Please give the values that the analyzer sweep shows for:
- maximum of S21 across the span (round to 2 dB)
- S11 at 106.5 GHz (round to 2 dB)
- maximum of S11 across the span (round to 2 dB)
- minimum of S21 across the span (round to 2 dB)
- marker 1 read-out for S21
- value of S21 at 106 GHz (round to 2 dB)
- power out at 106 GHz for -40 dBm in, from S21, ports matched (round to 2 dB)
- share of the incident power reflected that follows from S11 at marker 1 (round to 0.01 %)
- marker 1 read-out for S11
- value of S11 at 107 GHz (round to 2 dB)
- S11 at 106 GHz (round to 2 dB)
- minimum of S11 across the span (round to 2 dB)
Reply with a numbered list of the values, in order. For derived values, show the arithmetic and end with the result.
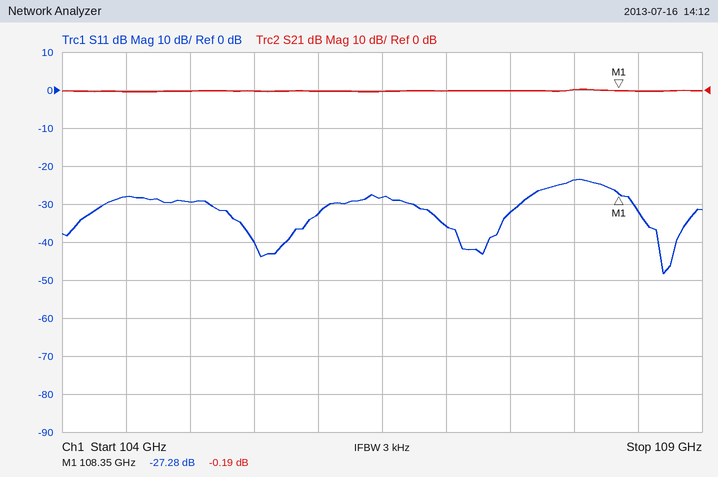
1. 0 dB
2. -28 dB
3. -24 dB
4. 0 dB
5. -0.19 dB
6. 0 dB
7. -40 dBm + (0 dB) = -40 dBm
8. 10^(-27.28/10) ≈ 0.19 %
9. -27.28 dB
10. -36 dB
11. -32 dB
12. -48 dB
